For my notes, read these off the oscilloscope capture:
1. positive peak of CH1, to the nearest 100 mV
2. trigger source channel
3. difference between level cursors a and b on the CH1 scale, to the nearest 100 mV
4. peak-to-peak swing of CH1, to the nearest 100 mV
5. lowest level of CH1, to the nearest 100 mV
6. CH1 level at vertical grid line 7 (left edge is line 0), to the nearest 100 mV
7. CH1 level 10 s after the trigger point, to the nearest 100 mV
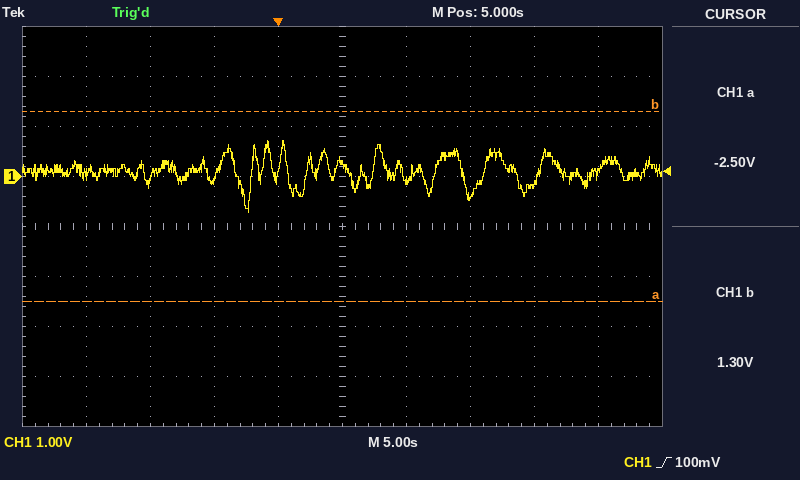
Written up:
700 mV
CH1
3.8 V
1.4 V
-700 mV
-400 mV
-100 mV
